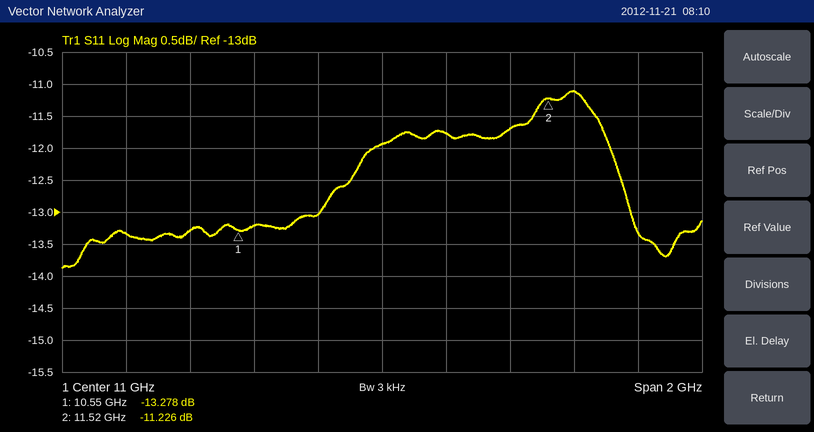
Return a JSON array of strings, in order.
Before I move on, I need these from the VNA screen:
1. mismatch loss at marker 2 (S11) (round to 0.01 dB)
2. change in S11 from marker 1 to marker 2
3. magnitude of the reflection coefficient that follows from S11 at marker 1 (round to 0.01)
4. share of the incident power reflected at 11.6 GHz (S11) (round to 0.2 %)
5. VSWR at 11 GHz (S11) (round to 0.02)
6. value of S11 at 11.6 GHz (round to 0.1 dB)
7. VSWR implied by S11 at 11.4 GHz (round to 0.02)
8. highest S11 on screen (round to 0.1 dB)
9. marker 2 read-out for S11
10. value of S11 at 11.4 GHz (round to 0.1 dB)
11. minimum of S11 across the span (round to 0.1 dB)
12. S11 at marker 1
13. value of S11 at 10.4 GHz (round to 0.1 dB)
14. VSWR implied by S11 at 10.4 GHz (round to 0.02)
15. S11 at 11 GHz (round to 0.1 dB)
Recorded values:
["0.34 dB", "2.052 dB", "0.22", "7.8 %", "1.68", "-11.1 dB", "1.70", "-11.1 dB", "-11.226 dB", "-11.7 dB", "-13.9 dB", "-13.278 dB", "-13.3 dB", "1.56", "-11.9 dB"]
